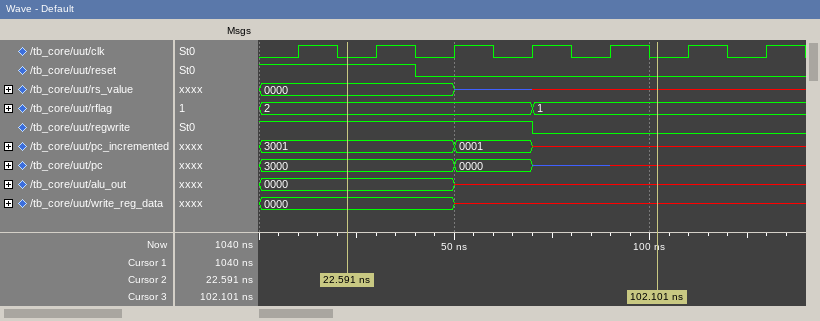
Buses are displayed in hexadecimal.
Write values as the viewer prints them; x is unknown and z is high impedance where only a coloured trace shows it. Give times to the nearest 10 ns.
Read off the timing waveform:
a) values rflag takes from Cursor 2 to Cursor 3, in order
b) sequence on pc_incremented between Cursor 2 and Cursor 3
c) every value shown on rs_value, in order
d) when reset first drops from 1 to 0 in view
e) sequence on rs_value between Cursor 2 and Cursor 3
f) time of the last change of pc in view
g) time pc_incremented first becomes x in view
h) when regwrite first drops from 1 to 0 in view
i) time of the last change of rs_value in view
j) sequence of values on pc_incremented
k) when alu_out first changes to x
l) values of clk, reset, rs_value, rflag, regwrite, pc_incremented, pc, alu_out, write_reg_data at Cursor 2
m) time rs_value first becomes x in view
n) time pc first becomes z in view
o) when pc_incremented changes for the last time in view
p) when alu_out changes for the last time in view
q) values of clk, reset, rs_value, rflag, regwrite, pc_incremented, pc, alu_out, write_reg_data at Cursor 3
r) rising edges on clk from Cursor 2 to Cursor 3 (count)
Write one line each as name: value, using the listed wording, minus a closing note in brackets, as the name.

values rflag takes from Cursor 2 to Cursor 3, in order: 2, 1
sequence on pc_incremented between Cursor 2 and Cursor 3: 3001, 0001, x
every value shown on rs_value, in order: 0000, z, x
when reset first drops from 1 to 0 in view: 40 ns
sequence on rs_value between Cursor 2 and Cursor 3: 0000, z, x
time of the last change of pc in view: 90 ns
time pc_incremented first becomes x in view: 70 ns
when regwrite first drops from 1 to 0 in view: 70 ns
time of the last change of rs_value in view: 70 ns
sequence of values on pc_incremented: 3001, 0001, x
when alu_out first changes to x: 50 ns
values of clk, reset, rs_value, rflag, regwrite, pc_incremented, pc, alu_out, write_reg_data at Cursor 2: clk=0, reset=1, rs_value=0000, rflag=2, regwrite=1, pc_incremented=3001, pc=3000, alu_out=0000, write_reg_data=0000
time rs_value first becomes x in view: 70 ns
time pc first becomes z in view: 70 ns
when pc_incremented changes for the last time in view: 70 ns
when alu_out changes for the last time in view: 50 ns
values of clk, reset, rs_value, rflag, regwrite, pc_incremented, pc, alu_out, write_reg_data at Cursor 3: clk=0, reset=0, rs_value=x, rflag=1, regwrite=0, pc_incremented=x, pc=x, alu_out=x, write_reg_data=x
rising edges on clk from Cursor 2 to Cursor 3: 4
